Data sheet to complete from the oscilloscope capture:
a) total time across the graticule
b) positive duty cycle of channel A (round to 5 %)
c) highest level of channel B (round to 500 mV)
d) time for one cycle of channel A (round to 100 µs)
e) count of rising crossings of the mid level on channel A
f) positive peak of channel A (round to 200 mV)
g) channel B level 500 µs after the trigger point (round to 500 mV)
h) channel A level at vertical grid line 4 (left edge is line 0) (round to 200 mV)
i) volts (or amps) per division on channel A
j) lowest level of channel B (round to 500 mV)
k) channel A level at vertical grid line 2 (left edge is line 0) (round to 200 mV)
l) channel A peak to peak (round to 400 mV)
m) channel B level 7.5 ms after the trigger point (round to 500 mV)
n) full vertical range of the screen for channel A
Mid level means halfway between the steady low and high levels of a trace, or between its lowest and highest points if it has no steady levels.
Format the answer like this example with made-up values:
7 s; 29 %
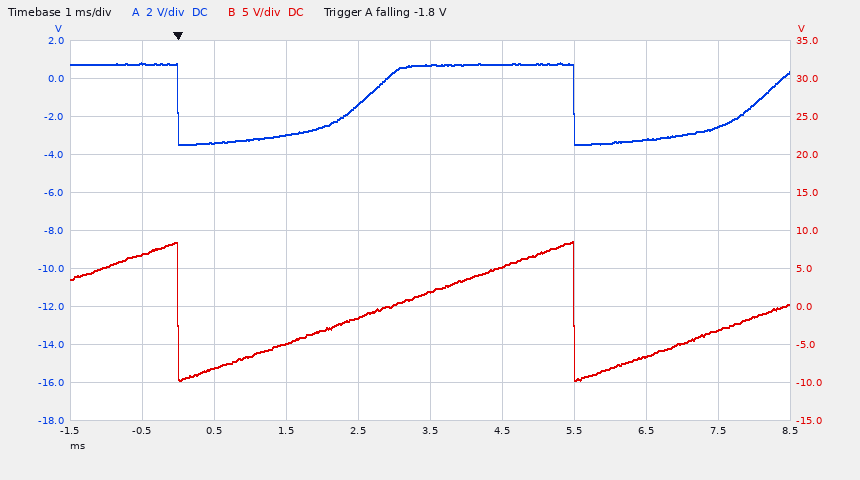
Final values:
10 ms; 55 %; 8.5 V; 5.5 ms; 2; 800 mV; -8.0 V; -1.4 V; 2 V; -9.5 V; -3.4 V; 4.4 V; -3.0 V; 20 V
